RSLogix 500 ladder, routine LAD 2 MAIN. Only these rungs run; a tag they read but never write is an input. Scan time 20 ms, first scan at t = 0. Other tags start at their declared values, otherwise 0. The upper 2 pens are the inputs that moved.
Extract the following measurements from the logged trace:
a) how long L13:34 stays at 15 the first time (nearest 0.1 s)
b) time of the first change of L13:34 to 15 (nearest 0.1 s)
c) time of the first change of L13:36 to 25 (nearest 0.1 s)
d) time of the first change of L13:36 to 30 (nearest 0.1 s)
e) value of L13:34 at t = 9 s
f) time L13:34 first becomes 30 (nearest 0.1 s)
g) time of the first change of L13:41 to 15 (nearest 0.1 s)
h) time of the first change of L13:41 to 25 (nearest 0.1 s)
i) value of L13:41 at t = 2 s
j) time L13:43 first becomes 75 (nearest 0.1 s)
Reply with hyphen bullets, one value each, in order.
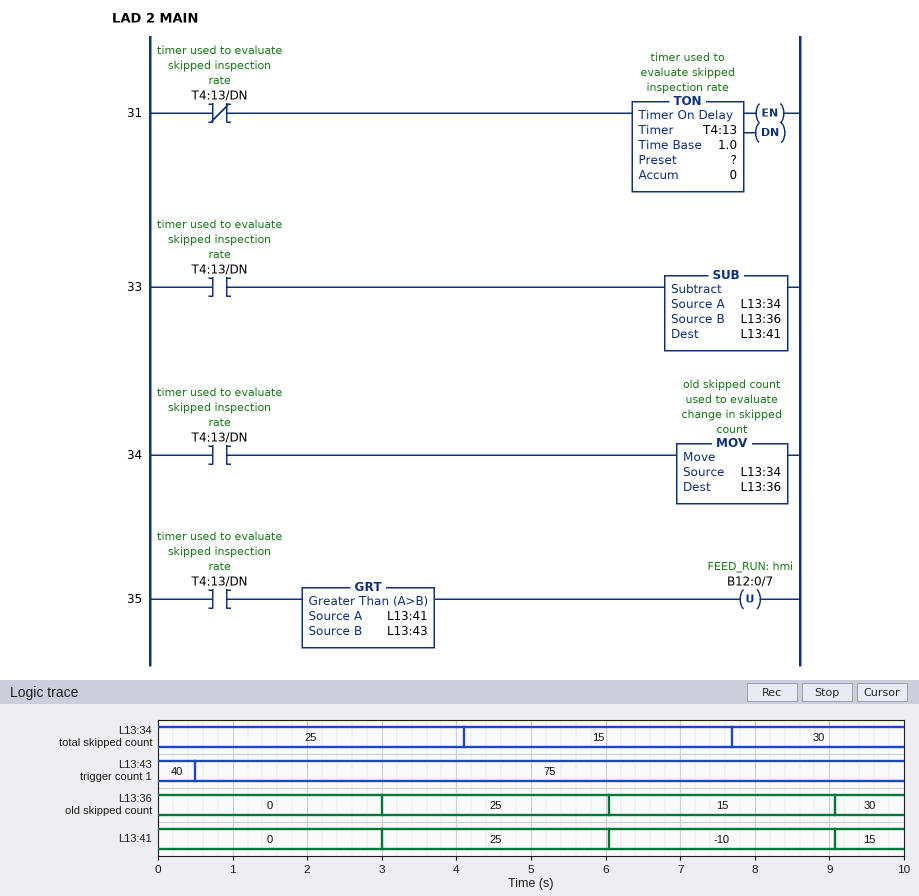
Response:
- 3.6 s
- 4.1 s
- 3.0 s
- 9.1 s
- 30
- 7.7 s
- 9.1 s
- 3.0 s
- 0
- 0.5 s
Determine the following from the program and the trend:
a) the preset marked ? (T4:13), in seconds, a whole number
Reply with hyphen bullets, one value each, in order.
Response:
- 3 s
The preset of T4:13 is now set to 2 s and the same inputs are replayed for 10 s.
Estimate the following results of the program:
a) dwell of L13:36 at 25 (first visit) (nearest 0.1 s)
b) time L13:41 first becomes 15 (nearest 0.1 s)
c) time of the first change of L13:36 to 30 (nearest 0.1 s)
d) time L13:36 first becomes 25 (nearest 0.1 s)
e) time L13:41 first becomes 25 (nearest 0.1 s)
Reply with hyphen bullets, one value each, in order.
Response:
- 4.1 s
- 8.1 s
- 8.1 s
- 2.0 s
- 2.0 s
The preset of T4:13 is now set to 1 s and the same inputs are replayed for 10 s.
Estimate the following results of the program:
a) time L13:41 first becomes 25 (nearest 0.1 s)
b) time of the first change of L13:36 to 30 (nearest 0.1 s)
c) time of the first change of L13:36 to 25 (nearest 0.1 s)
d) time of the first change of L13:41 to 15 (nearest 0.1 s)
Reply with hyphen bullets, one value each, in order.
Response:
- 1.0 s
- 8.3 s
- 1.0 s
- 8.3 s
